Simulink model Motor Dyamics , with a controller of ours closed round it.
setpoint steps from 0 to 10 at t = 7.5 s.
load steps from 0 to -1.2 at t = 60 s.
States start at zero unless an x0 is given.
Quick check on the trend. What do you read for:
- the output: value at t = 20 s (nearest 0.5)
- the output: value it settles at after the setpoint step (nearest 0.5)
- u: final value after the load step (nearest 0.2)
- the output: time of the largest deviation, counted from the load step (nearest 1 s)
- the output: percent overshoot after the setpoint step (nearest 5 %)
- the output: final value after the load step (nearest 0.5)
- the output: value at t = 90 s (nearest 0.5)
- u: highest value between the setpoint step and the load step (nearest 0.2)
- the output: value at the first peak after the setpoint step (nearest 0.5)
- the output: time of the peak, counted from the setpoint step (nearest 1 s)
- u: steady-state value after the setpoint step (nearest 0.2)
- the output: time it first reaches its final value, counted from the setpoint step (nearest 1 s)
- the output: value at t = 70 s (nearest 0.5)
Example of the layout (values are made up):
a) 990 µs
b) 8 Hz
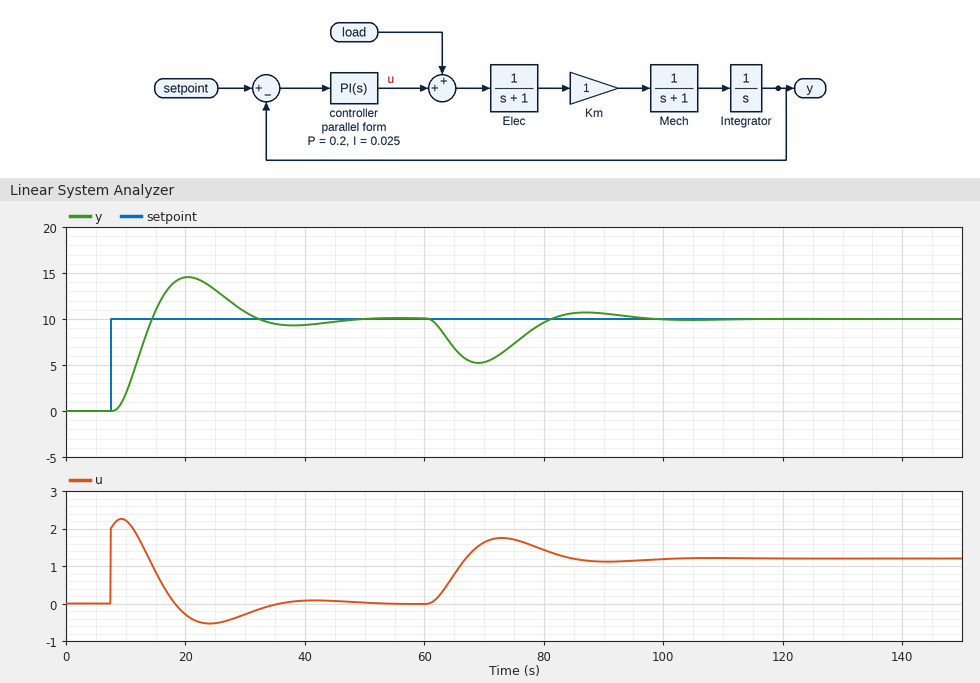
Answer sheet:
a) 14.5
b) 10.0
c) 1.2
d) 9 s
e) 45 %
f) 10.0
g) 10.5
h) 2.2
i) 14.5
j) 13 s
k) 0.0
l) 7 s
m) 5.5
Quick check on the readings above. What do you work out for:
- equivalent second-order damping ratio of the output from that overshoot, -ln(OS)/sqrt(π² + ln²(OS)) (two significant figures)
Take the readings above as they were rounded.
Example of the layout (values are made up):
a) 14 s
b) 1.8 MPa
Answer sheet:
a) 0.25
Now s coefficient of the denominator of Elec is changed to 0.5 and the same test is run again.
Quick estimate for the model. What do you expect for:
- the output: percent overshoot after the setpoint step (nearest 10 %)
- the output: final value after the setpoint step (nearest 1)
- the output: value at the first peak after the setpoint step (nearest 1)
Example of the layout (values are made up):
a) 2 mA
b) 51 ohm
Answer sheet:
a) 40 %
b) 10
c) 14
